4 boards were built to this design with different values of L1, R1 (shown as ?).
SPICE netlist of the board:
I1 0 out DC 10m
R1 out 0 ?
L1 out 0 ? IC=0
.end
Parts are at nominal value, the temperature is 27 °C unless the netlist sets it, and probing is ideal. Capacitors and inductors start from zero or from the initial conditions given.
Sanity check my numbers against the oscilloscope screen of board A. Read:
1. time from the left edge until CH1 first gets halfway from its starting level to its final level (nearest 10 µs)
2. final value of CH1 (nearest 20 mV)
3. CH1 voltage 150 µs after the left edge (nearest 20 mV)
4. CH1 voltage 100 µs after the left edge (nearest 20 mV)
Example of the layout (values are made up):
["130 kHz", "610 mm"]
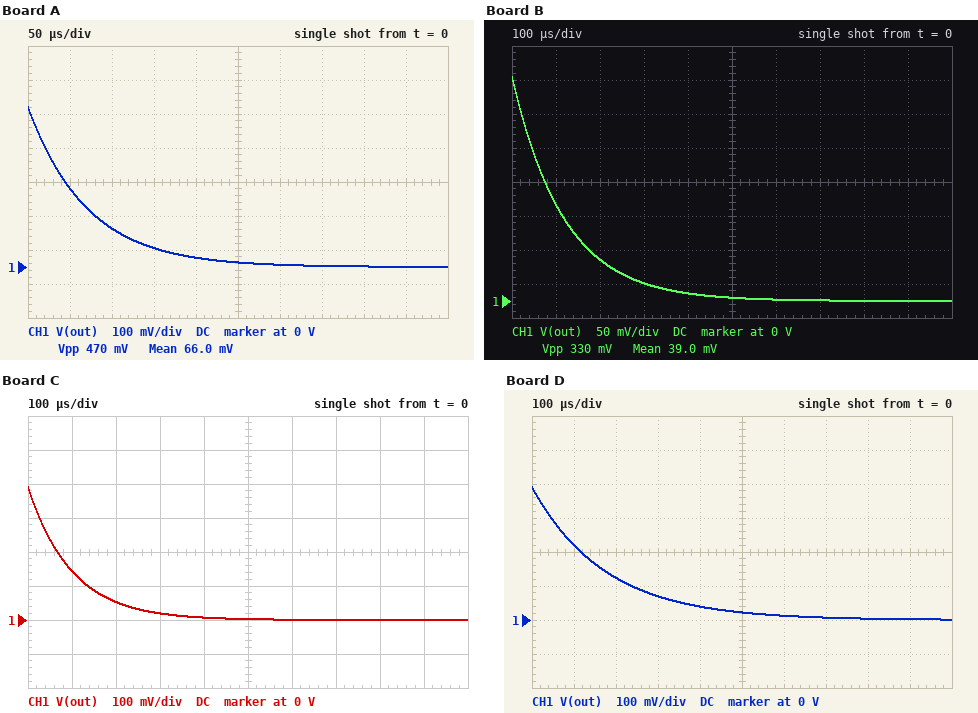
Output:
["50 µs", "0 V", "60 mV", "120 mV"]
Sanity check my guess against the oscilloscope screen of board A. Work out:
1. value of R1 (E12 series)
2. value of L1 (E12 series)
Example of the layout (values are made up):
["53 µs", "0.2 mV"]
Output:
["47 Ω", "3.3 mH"]
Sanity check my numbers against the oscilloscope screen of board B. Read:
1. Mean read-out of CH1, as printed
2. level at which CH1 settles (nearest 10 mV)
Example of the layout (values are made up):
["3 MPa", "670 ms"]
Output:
["39.0 mV", "0 V"]
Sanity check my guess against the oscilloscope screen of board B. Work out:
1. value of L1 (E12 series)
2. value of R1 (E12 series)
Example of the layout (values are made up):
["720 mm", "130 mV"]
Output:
["3.9 mH", "33 Ω"]
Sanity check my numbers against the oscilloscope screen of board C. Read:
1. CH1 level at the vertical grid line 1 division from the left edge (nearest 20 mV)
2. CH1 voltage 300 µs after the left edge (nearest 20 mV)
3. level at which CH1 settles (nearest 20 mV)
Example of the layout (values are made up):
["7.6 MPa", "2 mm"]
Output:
["140 mV", "20 mV", "0 V"]
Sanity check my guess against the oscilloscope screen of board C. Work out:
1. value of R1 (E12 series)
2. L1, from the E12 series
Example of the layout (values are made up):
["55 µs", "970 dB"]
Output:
["39 Ω", "3.9 mH"]
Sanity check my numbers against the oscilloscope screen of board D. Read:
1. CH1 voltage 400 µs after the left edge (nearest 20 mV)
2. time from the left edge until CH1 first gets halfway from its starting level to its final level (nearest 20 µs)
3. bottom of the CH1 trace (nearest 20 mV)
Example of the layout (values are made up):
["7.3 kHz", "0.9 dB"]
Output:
["40 mV", "120 µs", "0 V"]
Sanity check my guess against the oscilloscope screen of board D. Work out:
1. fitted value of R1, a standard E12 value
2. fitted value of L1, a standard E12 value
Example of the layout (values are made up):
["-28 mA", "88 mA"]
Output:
["39 Ω", "6.8 mH"]
